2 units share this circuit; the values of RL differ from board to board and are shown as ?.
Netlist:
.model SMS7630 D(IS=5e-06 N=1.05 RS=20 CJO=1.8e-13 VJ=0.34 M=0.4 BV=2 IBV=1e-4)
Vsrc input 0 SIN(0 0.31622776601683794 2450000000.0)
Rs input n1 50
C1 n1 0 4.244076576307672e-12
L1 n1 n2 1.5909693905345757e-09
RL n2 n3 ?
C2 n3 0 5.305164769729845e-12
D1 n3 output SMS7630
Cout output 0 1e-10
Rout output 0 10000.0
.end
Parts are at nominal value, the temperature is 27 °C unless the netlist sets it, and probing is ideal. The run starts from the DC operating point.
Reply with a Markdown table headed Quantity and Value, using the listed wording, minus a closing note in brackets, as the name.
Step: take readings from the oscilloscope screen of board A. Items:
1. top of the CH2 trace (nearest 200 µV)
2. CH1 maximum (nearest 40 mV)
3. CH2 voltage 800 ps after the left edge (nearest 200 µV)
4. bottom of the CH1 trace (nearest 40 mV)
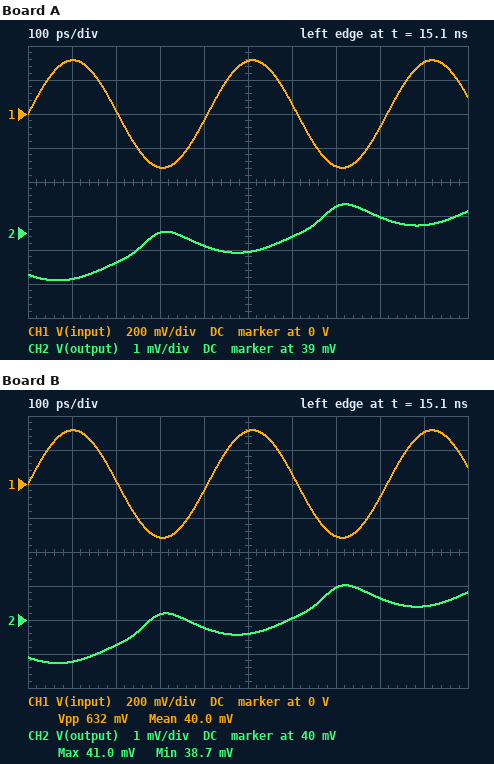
| Quantity | Value |
|---|---|
| top of the CH2 trace | 39.8 mV |
| CH1 maximum | 320 mV |
| CH2 voltage 800 ps after the left edge | 39.4 mV |
| bottom of the CH1 trace | -320 mV |
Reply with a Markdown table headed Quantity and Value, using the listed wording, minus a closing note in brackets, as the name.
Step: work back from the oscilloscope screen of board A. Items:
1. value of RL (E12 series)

| Quantity | Value |
|---|---|
| value of RL | 0.22 Ω |
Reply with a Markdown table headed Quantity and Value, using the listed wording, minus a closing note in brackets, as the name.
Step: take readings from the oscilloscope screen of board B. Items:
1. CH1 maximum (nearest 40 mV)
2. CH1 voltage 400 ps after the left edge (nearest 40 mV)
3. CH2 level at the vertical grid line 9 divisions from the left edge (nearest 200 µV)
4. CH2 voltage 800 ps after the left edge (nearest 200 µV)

| Quantity | Value |
|---|---|
| CH1 maximum | 320 mV |
| CH1 voltage 400 ps after the left edge | -40 mV |
| CH2 level at the vertical grid line 9 divisions from the left edge | 40.4 mV |
| CH2 voltage 800 ps after the left edge | 40.6 mV |
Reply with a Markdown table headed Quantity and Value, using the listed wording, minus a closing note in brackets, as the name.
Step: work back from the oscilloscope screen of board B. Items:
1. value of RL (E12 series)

| Quantity | Value |
|---|---|
| value of RL | 0.15 Ω |
